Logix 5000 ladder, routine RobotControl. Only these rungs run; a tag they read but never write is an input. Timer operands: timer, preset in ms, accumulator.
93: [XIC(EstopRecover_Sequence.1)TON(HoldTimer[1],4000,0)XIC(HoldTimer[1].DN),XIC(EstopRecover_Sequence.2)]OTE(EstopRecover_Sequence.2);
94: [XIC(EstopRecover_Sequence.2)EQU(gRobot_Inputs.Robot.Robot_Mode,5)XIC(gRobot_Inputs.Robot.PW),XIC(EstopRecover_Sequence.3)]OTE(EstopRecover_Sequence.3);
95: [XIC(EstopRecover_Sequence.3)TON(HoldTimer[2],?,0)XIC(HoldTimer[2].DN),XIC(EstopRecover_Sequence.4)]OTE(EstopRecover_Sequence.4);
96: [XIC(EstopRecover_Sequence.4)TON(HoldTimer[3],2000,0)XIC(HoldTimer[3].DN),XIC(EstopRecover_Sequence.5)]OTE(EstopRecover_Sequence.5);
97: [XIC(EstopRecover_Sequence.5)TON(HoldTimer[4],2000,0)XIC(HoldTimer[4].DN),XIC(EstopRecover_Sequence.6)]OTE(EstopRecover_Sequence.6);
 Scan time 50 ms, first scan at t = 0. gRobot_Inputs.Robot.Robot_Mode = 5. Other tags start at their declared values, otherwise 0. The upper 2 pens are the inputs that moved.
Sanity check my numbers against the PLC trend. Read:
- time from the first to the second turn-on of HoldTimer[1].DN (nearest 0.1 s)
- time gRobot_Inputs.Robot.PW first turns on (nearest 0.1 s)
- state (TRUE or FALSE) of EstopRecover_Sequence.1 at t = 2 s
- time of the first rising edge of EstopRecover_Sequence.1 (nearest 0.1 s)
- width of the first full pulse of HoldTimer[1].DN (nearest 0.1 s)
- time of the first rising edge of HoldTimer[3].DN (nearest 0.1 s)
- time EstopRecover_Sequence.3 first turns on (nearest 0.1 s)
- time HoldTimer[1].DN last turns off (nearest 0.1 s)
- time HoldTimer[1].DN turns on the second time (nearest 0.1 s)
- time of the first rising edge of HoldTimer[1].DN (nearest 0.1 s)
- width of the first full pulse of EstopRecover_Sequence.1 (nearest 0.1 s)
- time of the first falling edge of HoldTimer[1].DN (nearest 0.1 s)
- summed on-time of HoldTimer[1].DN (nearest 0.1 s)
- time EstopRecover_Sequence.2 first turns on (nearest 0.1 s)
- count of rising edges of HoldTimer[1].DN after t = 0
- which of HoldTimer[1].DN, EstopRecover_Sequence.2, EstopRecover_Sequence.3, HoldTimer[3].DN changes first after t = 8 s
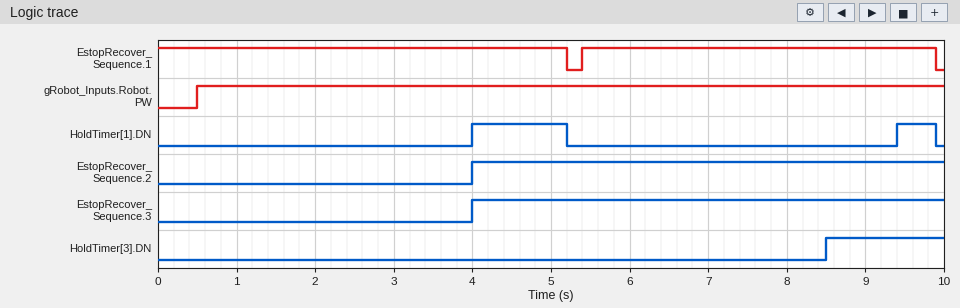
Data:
5.4 s
0.5 s
TRUE
5.4 s
1.2 s
8.5 s
4.0 s
9.9 s
9.4 s
4.0 s
4.5 s
5.2 s
1.7 s
4.0 s
2
HoldTimer[3].DN
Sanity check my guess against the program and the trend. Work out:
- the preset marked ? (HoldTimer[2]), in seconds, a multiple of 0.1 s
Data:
2.5 s
